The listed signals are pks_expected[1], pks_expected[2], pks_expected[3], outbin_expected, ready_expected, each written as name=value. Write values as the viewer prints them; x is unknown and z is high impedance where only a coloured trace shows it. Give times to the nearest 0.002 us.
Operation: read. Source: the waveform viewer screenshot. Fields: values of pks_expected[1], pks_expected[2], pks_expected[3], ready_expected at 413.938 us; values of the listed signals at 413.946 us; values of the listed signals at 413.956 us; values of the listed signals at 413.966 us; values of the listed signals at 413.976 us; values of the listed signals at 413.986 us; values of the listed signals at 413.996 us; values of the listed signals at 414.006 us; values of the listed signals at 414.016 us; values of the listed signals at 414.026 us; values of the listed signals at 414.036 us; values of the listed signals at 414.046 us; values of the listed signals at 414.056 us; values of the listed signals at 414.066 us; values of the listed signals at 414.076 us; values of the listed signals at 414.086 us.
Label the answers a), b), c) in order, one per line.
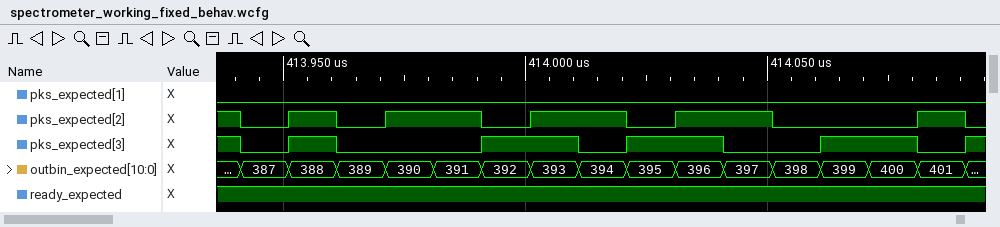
a) pks_expected[1]=0, pks_expected[2]=1, pks_expected[3]=1, ready_expected=1
b) pks_expected[1]=0, pks_expected[2]=0, pks_expected[3]=0, outbin_expected=387, ready_expected=1
c) pks_expected[1]=0, pks_expected[2]=1, pks_expected[3]=1, outbin_expected=388, ready_expected=1
d) pks_expected[1]=0, pks_expected[2]=0, pks_expected[3]=0, outbin_expected=389, ready_expected=1
e) pks_expected[1]=0, pks_expected[2]=1, pks_expected[3]=0, outbin_expected=390, ready_expected=1
f) pks_expected[1]=0, pks_expected[2]=1, pks_expected[3]=0, outbin_expected=391, ready_expected=1
g) pks_expected[1]=0, pks_expected[2]=0, pks_expected[3]=1, outbin_expected=392, ready_expected=1
h) pks_expected[1]=0, pks_expected[2]=1, pks_expected[3]=1, outbin_expected=393, ready_expected=1
i) pks_expected[1]=0, pks_expected[2]=1, pks_expected[3]=0, outbin_expected=394, ready_expected=1
j) pks_expected[1]=0, pks_expected[2]=0, pks_expected[3]=1, outbin_expected=395, ready_expected=1
k) pks_expected[1]=0, pks_expected[2]=1, pks_expected[3]=1, outbin_expected=396, ready_expected=1
l) pks_expected[1]=0, pks_expected[2]=1, pks_expected[3]=0, outbin_expected=397, ready_expected=1
m) pks_expected[1]=0, pks_expected[2]=0, pks_expected[3]=0, outbin_expected=398, ready_expected=1
n) pks_expected[1]=0, pks_expected[2]=0, pks_expected[3]=1, outbin_expected=399, ready_expected=1
o) pks_expected[1]=0, pks_expected[2]=0, pks_expected[3]=1, outbin_expected=400, ready_expected=1
p) pks_expected[1]=0, pks_expected[2]=1, pks_expected[3]=0, outbin_expected=401, ready_expected=1
